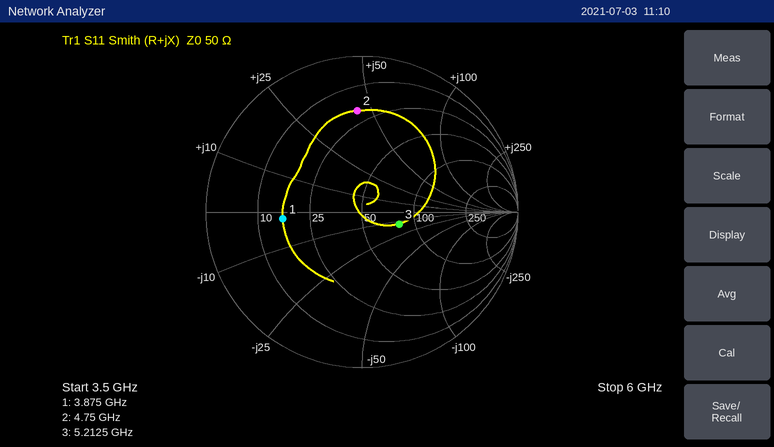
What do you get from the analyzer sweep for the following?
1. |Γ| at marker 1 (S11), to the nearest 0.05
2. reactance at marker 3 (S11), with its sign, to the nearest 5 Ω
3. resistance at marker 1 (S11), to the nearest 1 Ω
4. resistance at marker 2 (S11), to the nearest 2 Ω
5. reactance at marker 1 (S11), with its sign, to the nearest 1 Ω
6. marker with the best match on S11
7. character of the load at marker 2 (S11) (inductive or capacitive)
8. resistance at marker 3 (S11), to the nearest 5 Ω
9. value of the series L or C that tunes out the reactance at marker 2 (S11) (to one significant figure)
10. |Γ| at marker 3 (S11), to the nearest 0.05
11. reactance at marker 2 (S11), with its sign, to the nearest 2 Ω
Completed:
0.50
-15 Ω
16 Ω
20 Ω
-2 Ω
marker 3
inductive
80 Ω
800 fF
0.25
+44 Ω
